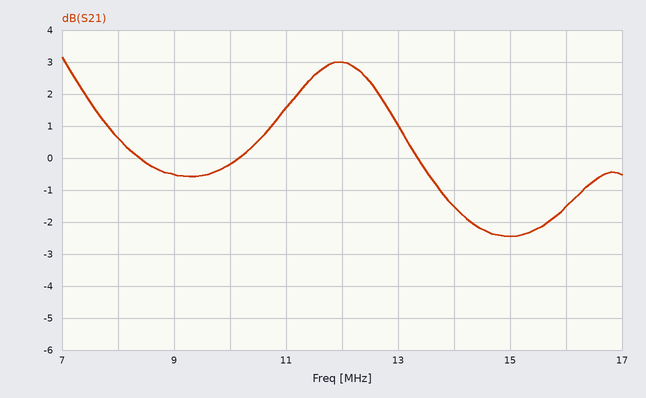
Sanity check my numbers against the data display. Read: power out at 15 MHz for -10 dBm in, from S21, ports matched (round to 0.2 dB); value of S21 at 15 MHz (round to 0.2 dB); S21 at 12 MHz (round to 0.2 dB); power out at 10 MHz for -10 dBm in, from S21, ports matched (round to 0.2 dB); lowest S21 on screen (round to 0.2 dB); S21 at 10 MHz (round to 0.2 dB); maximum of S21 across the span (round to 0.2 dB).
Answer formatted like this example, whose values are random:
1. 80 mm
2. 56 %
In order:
1. -12.4 dBm
2. -2.4 dB
3. 3.0 dB
4. -10.2 dBm
5. -2.4 dB
6. -0.2 dB
7. 3.2 dB
